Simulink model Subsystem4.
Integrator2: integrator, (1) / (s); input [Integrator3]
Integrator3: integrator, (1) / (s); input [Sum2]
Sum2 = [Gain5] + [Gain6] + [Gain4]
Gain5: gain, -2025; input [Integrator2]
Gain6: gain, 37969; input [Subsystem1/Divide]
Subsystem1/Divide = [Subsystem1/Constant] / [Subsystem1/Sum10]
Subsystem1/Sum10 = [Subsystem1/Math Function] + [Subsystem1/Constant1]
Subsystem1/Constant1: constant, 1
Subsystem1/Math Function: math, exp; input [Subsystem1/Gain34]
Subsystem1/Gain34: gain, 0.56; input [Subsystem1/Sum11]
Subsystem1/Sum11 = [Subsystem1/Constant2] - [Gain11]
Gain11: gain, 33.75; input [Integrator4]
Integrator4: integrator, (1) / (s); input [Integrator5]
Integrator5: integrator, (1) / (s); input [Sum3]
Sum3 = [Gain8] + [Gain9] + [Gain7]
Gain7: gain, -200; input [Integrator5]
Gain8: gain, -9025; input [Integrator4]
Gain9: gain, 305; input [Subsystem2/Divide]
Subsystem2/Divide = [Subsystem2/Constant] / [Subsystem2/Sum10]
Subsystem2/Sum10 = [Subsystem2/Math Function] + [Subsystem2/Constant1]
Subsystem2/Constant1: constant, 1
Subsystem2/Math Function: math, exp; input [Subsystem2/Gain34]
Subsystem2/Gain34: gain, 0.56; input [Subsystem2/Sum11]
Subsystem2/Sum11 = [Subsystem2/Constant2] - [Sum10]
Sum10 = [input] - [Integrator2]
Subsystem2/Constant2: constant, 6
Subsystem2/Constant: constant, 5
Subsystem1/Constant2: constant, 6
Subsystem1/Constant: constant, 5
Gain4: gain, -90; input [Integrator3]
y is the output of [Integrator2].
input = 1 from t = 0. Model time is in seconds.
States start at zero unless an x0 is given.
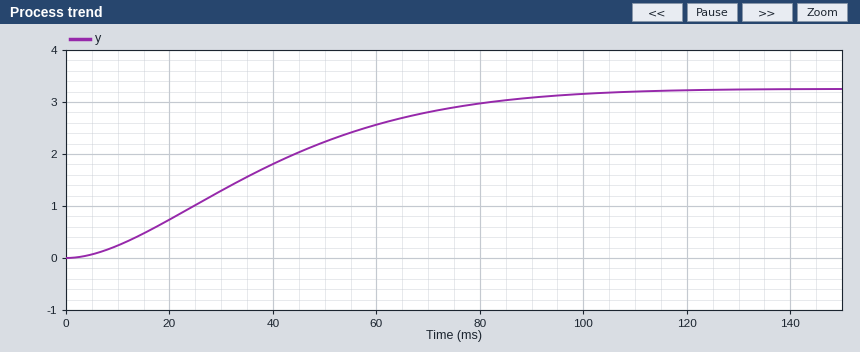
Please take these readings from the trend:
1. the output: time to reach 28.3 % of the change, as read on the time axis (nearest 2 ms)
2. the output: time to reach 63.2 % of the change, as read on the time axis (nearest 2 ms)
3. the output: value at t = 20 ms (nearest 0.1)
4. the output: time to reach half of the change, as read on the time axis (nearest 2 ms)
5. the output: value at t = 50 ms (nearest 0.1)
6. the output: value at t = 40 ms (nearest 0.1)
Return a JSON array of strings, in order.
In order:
["24 ms", "46 ms", "0.7", "36 ms", "2.2", "1.8"]
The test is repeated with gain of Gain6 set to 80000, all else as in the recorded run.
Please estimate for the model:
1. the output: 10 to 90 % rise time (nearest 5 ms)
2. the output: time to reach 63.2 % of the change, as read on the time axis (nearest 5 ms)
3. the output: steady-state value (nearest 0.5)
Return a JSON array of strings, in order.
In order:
["65 ms", "45 ms", "6.5"]
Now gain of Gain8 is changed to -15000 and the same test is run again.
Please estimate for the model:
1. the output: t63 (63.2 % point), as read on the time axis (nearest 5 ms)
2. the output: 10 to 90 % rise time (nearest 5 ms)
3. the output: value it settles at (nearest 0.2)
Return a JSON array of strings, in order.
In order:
["45 ms", "70 ms", "3.2"]
